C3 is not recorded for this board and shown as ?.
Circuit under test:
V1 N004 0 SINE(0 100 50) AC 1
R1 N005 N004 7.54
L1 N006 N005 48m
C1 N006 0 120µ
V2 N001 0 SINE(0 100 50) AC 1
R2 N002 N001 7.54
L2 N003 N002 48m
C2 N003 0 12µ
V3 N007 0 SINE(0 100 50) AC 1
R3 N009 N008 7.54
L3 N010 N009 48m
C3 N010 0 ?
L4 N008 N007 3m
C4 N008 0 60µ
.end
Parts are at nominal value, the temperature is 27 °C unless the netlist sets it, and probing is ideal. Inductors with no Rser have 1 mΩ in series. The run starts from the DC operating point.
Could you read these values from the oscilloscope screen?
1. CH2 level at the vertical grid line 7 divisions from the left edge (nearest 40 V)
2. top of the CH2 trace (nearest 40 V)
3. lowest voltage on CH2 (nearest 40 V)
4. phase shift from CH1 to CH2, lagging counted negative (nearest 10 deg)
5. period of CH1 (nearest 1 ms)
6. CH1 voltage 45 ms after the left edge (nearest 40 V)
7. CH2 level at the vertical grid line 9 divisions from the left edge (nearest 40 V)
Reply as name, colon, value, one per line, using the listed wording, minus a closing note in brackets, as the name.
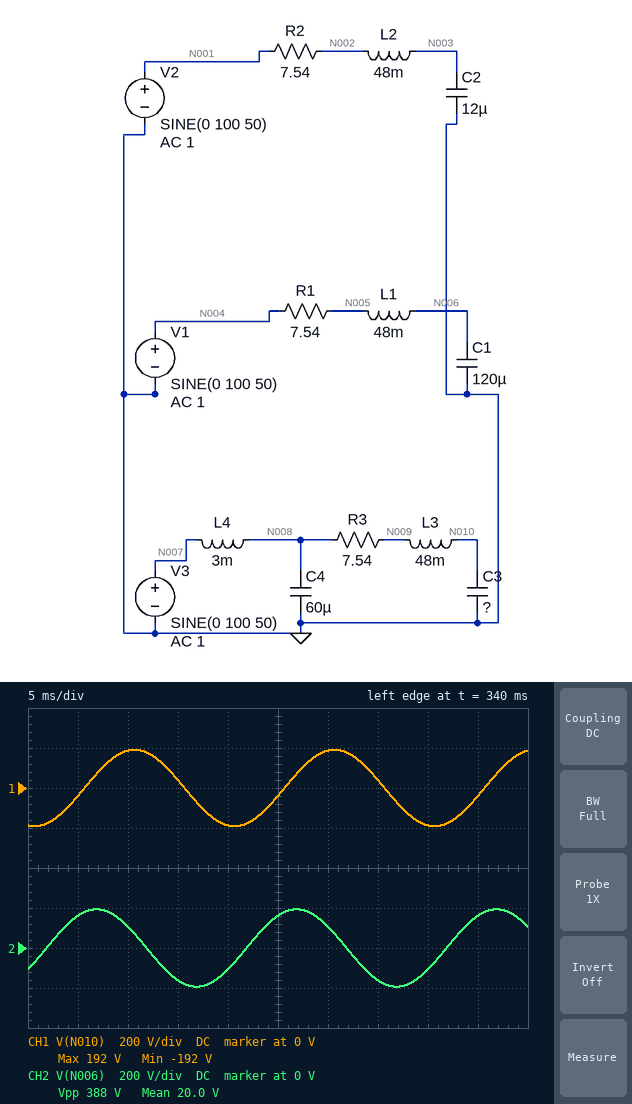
CH2 level at the vertical grid line 7 divisions from the left edge: -160 V
top of the CH2 trace: 200 V
lowest voltage on CH2: -200 V
phase shift from CH1 to CH2, lagging counted negative: 70 deg
period of CH1: 20 ms
CH1 voltage 45 ms after the left edge: -40 V
CH2 level at the vertical grid line 9 divisions from the left edge: 160 V
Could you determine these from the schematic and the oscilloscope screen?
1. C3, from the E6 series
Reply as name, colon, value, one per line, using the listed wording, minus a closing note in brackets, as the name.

C3, from the E6 series: 220 µF
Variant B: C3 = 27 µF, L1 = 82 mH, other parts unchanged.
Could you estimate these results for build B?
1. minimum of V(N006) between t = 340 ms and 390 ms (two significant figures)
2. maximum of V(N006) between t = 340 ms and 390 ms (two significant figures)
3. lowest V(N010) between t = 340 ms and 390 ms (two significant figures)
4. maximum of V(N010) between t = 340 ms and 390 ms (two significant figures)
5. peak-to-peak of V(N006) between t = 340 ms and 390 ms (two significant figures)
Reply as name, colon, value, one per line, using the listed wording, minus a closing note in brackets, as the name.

minimum of V(N006) between t = 340 ms and 390 ms: -350 V
maximum of V(N006) between t = 340 ms and 390 ms: 350 V
lowest V(N010) between t = 340 ms and 390 ms: -120 V
maximum of V(N010) between t = 340 ms and 390 ms: 120 V
peak-to-peak of V(N006) between t = 340 ms and 390 ms: 700 V
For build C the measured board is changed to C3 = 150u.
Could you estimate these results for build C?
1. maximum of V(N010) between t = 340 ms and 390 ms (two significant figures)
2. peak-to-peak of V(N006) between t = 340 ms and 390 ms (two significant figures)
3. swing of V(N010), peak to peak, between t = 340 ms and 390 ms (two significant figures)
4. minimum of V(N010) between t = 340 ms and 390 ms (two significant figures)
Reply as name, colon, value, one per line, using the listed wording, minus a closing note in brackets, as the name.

maximum of V(N010) between t = 340 ms and 390 ms: 240 V
peak-to-peak of V(N006) between t = 340 ms and 390 ms: 390 V
swing of V(N010), peak to peak, between t = 340 ms and 390 ms: 470 V
minimum of V(N010) between t = 340 ms and 390 ms: -240 V
